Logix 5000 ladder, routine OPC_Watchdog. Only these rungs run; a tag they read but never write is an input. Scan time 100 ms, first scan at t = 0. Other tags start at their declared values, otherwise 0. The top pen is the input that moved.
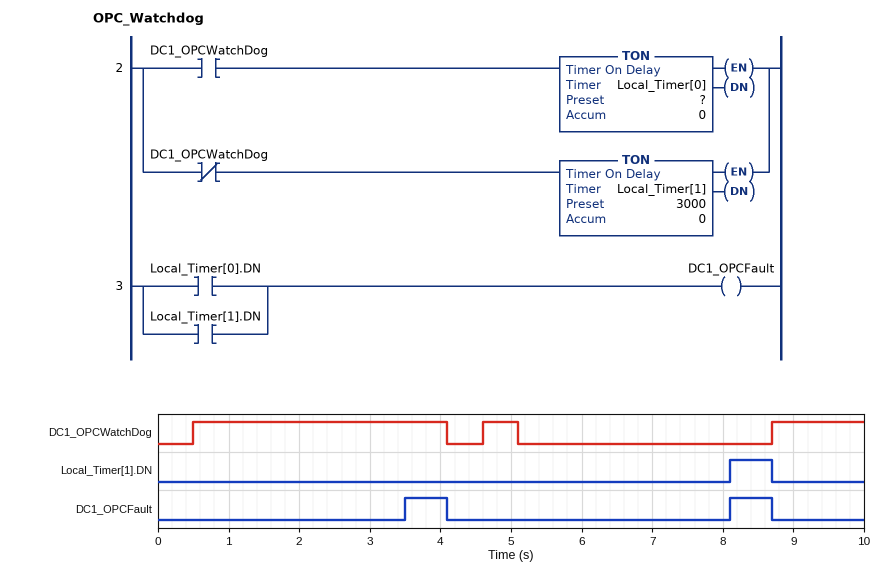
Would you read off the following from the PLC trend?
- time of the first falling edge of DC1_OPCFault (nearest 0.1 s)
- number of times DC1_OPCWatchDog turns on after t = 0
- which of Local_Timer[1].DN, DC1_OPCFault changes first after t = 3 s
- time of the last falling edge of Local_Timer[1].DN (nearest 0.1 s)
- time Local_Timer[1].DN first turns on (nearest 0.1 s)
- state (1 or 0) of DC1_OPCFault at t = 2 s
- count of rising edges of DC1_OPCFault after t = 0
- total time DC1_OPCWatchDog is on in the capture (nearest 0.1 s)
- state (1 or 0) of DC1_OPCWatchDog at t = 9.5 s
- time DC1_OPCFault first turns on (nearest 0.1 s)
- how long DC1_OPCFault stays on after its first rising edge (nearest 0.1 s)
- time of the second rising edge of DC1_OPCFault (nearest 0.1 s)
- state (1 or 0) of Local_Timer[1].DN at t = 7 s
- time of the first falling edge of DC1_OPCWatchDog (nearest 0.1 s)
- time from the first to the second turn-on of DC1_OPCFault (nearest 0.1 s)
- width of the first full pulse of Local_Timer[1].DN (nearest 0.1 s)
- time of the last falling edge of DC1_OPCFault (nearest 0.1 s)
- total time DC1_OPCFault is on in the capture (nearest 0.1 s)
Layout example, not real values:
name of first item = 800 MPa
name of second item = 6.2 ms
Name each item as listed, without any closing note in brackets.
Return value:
time of the first falling edge of DC1_OPCFault = 4.1 s
number of times DC1_OPCWatchDog turns on after t = 0 = 3
which of Local_Timer[1].DN, DC1_OPCFault changes first after t = 3 s = DC1_OPCFault
time of the last falling edge of Local_Timer[1].DN = 8.7 s
time Local_Timer[1].DN first turns on = 8.1 s
state (1 or 0) of DC1_OPCFault at t = 2 s = 0
count of rising edges of DC1_OPCFault after t = 0 = 2
total time DC1_OPCWatchDog is on in the capture = 5.4 s
state (1 or 0) of DC1_OPCWatchDog at t = 9.5 s = 1
time DC1_OPCFault first turns on = 3.5 s
how long DC1_OPCFault stays on after its first rising edge = 0.6 s
time of the second rising edge of DC1_OPCFault = 8.1 s
state (1 or 0) of Local_Timer[1].DN at t = 7 s = 0
time of the first falling edge of DC1_OPCWatchDog = 4.1 s
time from the first to the second turn-on of DC1_OPCFault = 4.6 s
width of the first full pulse of Local_Timer[1].DN = 0.6 s
time of the last falling edge of DC1_OPCFault = 8.7 s
total time DC1_OPCFault is on in the capture = 1.2 s
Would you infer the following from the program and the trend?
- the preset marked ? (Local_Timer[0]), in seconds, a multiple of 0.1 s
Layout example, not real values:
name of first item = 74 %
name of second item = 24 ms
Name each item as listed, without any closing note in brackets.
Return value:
the preset marked ? (Local_Timer[0]), in seconds, a multiple of 0.1 s = 3.0 s
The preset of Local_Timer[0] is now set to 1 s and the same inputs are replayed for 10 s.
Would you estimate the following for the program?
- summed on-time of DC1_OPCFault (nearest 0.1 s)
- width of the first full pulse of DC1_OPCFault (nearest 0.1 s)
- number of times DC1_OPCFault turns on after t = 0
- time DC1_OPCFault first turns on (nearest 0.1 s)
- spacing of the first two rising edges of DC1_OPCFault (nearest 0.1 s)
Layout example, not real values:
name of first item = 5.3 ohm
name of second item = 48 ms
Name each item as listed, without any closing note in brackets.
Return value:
summed on-time of DC1_OPCFault = 3.5 s
width of the first full pulse of DC1_OPCFault = 2.6 s
number of times DC1_OPCFault turns on after t = 0 = 3
time DC1_OPCFault first turns on = 1.5 s
spacing of the first two rising edges of DC1_OPCFault = 6.6 s
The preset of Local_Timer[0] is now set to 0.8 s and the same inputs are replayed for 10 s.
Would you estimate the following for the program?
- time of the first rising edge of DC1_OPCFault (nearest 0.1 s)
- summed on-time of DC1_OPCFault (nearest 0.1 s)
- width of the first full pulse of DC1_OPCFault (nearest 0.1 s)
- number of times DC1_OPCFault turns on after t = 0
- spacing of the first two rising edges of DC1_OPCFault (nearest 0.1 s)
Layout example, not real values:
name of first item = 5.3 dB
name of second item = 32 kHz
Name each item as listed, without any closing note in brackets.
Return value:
time of the first rising edge of DC1_OPCFault = 1.3 s
summed on-time of DC1_OPCFault = 3.9 s
width of the first full pulse of DC1_OPCFault = 2.8 s
number of times DC1_OPCFault turns on after t = 0 = 3
spacing of the first two rising edges of DC1_OPCFault = 6.8 s
